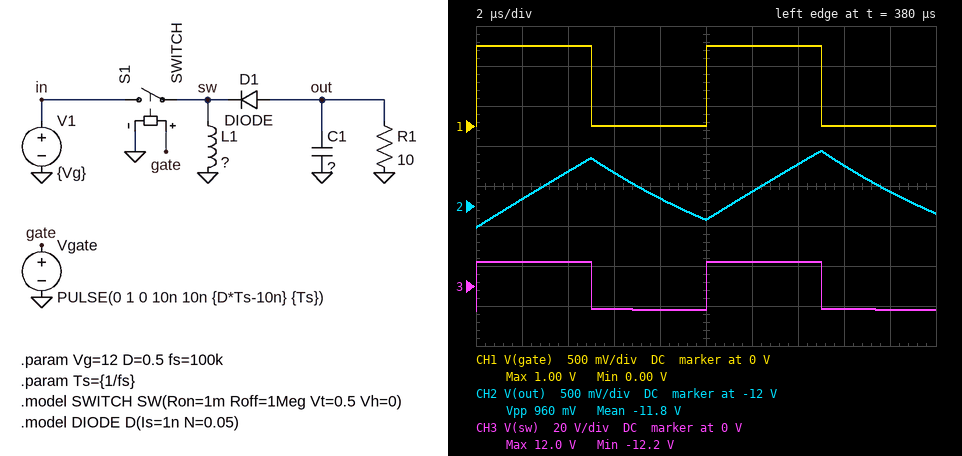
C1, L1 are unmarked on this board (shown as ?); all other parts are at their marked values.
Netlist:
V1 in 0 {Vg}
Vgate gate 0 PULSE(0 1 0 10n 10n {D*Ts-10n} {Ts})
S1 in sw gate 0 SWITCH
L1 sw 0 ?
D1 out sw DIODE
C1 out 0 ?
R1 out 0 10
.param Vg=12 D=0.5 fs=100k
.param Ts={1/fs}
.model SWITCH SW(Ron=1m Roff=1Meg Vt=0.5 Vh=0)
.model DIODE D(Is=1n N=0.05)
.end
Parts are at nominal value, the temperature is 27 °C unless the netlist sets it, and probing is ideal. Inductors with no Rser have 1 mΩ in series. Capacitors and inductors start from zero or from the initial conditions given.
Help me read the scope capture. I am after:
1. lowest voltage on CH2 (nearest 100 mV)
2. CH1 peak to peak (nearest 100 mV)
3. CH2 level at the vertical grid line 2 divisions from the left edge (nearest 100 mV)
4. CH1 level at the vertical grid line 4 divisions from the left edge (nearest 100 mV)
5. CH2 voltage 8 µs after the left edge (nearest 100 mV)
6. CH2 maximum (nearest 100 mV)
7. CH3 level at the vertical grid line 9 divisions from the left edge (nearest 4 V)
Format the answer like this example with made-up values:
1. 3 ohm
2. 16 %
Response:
1. -12.3 V
2. 1.0 V
3. -11.6 V
4. 0 V
5. -11.9 V
6. -11.3 V
7. -12 V
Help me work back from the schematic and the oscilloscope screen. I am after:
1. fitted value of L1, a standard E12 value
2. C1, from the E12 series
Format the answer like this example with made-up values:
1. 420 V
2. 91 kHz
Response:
1. 150 µH
2. 6.8 µF
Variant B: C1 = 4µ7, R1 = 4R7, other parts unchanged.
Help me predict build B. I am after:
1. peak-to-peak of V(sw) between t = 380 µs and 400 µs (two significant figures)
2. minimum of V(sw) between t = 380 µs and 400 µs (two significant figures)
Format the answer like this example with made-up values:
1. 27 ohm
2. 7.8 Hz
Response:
1. 25 V
2. -13 V
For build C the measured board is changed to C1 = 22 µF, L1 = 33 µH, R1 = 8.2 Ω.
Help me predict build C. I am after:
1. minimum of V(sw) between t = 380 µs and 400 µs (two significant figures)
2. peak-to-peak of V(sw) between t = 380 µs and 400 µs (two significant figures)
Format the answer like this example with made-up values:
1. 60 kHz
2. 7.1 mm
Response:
1. -10 V
2. 22 V
